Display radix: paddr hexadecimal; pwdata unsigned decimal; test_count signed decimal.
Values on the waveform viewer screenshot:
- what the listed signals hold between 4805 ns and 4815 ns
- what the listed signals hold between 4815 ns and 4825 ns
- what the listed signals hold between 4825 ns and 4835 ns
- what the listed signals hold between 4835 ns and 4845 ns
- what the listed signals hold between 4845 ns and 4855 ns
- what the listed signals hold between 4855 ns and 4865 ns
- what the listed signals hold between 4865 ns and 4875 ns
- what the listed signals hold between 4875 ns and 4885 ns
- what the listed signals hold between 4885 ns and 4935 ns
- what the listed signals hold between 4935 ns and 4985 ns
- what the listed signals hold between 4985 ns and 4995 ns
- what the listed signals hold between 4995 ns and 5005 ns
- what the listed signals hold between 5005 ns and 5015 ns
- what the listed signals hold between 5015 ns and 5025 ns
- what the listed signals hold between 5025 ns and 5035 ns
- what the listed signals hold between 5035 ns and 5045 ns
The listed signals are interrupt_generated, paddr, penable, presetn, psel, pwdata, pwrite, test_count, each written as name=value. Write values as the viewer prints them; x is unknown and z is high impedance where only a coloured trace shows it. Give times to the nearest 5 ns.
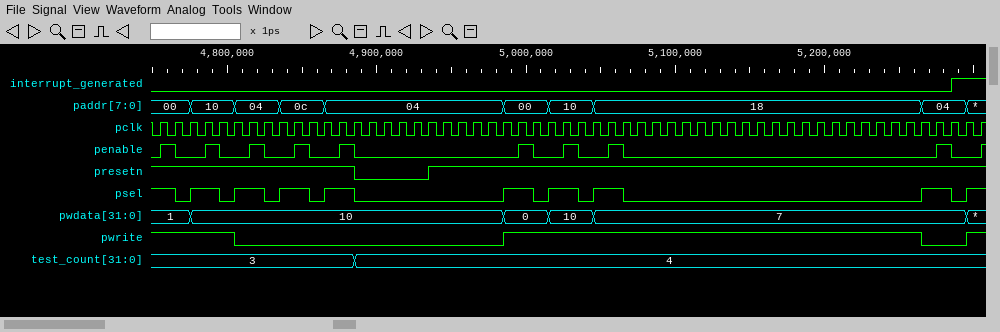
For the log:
interrupt_generated=0, paddr=04, penable=0, presetn=1, psel=1, pwdata=10, pwrite=0, test_count=3
interrupt_generated=0, paddr=04, penable=1, presetn=1, psel=1, pwdata=10, pwrite=0, test_count=3
interrupt_generated=0, paddr=04, penable=0, presetn=1, psel=0, pwdata=10, pwrite=0, test_count=3
interrupt_generated=0, paddr=0c, penable=0, presetn=1, psel=1, pwdata=10, pwrite=0, test_count=3
interrupt_generated=0, paddr=0c, penable=1, presetn=1, psel=1, pwdata=10, pwrite=0, test_count=3
interrupt_generated=0, paddr=0c, penable=0, presetn=1, psel=0, pwdata=10, pwrite=0, test_count=3
interrupt_generated=0, paddr=04, penable=0, presetn=1, psel=1, pwdata=10, pwrite=0, test_count=3
interrupt_generated=0, paddr=04, penable=1, presetn=1, psel=1, pwdata=10, pwrite=0, test_count=3
interrupt_generated=0, paddr=04, penable=0, presetn=0, psel=0, pwdata=10, pwrite=0, test_count=4
interrupt_generated=0, paddr=04, penable=0, presetn=1, psel=0, pwdata=10, pwrite=0, test_count=4
interrupt_generated=0, paddr=00, penable=0, presetn=1, psel=1, pwdata=0, pwrite=1, test_count=4
interrupt_generated=0, paddr=00, penable=1, presetn=1, psel=1, pwdata=0, pwrite=1, test_count=4
interrupt_generated=0, paddr=00, penable=0, presetn=1, psel=0, pwdata=0, pwrite=1, test_count=4
interrupt_generated=0, paddr=10, penable=0, presetn=1, psel=1, pwdata=10, pwrite=1, test_count=4
interrupt_generated=0, paddr=10, penable=1, presetn=1, psel=1, pwdata=10, pwrite=1, test_count=4
interrupt_generated=0, paddr=10, penable=0, presetn=1, psel=0, pwdata=10, pwrite=1, test_count=4
